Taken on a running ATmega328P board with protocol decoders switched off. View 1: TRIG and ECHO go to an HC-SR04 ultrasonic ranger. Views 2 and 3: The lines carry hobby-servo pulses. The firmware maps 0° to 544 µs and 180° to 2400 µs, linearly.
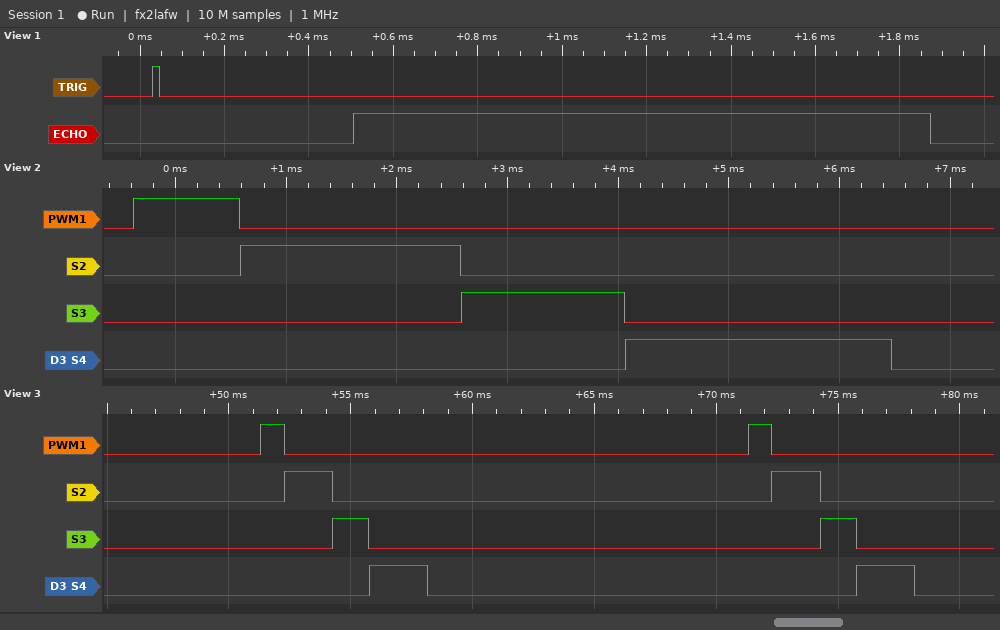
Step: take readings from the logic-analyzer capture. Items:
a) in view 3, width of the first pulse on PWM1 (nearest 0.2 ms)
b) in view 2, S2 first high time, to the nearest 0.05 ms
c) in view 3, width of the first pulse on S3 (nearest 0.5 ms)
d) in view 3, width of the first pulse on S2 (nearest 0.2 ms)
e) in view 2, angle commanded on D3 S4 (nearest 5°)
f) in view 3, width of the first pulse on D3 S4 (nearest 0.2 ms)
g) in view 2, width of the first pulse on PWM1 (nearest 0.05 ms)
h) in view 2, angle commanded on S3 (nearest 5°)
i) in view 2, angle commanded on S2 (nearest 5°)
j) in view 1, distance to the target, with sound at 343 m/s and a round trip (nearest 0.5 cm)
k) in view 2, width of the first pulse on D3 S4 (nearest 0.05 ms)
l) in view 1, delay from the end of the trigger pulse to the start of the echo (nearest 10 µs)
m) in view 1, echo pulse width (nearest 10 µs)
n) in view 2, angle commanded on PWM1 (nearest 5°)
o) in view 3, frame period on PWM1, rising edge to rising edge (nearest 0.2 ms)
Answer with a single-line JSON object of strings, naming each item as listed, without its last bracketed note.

{"in view 3, width of the first pulse on PWM1": "1.0 ms", "in view 2, S2 first high time, to the nearest 0.05 ms": "2.00 ms", "in view 3, width of the first pulse on S3": "1.5 ms", "in view 3, width of the first pulse on S2": "2.0 ms", "in view 2, angle commanded on D3 S4": "180°", "in view 3, width of the first pulse on D3 S4": "2.4 ms", "in view 2, width of the first pulse on PWM1": "0.95 ms", "in view 2, angle commanded on S3": "90°", "in view 2, angle commanded on S2": "140°", "in view 1, distance to the target, with sound at 343 m/s and a round trip": "23.5 cm", "in view 2, width of the first pulse on D3 S4": "2.40 ms", "in view 1, delay from the end of the trigger pulse to the start of the echo": "460 µs", "in view 1, echo pulse width": "1370 µs", "in view 2, angle commanded on PWM1": "40°", "in view 3, frame period on PWM1, rising edge to rising edge": "20.0 ms"}
